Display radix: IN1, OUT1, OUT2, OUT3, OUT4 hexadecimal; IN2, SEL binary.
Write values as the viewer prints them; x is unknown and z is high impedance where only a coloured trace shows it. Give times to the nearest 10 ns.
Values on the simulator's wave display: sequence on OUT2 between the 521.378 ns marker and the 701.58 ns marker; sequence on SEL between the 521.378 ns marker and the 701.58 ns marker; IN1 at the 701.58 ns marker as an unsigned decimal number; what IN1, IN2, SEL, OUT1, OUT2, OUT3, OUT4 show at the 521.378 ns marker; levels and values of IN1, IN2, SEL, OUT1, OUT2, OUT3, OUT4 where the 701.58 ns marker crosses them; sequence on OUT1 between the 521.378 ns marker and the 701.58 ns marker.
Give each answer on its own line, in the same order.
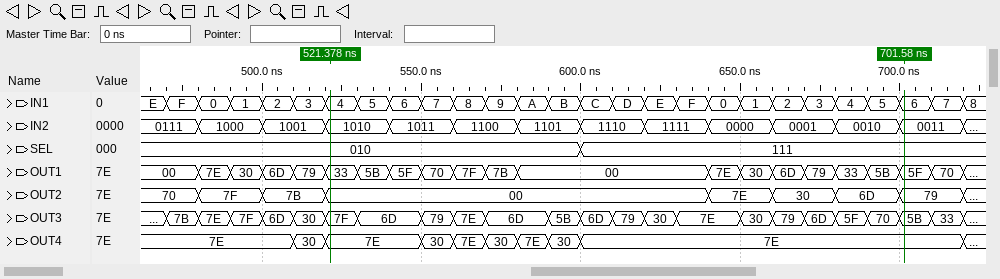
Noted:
00, 7E, 30, 6D, 79
010, 111
6
IN1=4, IN2=1010, SEL=010, OUT1=33, OUT2=00, OUT3=7F, OUT4=7E
IN1=6, IN2=0011, SEL=111, OUT1=5F, OUT2=79, OUT3=5B, OUT4=7E
33, 5B, 5F, 70, 7F, 7B, 00, 7E, 30, 6D, 79, 33, 5B, 5F
